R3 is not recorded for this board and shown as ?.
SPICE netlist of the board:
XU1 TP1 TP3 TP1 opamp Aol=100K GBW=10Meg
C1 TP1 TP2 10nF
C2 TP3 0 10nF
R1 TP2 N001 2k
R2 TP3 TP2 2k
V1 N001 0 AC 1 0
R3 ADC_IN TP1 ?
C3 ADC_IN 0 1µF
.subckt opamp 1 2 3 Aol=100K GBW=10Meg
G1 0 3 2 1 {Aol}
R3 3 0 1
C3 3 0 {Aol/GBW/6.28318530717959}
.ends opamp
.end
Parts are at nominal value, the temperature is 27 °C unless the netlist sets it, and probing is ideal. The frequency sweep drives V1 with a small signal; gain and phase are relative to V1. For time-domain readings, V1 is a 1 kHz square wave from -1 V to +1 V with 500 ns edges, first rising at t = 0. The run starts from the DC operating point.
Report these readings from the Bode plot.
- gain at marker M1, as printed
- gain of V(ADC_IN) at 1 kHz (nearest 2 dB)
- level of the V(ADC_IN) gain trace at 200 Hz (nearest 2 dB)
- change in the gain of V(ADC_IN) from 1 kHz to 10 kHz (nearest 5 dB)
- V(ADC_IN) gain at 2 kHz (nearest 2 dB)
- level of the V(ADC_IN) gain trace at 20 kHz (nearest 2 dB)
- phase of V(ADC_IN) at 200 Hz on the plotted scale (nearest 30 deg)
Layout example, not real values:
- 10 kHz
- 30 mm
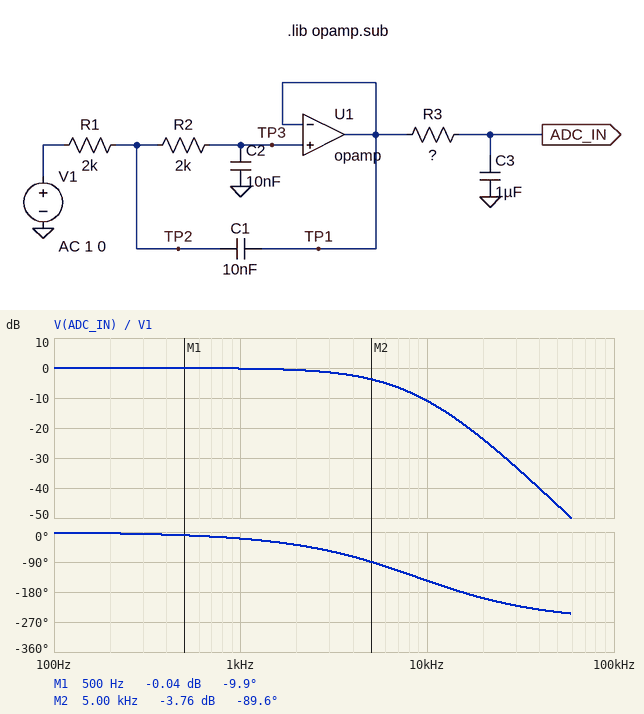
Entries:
- -0.04 dB
- 0 dB
- 0 dB
- -10 dB
- 0 dB
- -24 dB
- 0 deg
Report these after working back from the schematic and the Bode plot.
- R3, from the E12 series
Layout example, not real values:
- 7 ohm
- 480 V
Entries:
- 15 Ω
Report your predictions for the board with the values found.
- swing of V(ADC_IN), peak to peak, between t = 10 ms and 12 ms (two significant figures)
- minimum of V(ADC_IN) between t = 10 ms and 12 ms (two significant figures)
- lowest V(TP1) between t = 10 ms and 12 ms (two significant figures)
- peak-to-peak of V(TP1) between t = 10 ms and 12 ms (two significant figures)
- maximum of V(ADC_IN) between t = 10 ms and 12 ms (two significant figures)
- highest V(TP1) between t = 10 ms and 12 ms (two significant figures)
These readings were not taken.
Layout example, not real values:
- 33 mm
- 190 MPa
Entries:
- 2.0 V
- -1.0 V
- -1.0 V
- 2.0 V
- 1.0 V
- 1.0 V
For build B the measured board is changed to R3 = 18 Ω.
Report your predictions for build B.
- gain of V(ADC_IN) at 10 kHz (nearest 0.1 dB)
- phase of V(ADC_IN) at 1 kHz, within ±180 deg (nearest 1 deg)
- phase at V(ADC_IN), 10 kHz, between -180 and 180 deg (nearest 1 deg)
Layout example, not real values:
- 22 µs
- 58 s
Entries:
- -11.8 dB
- -21 deg
- -152 deg
